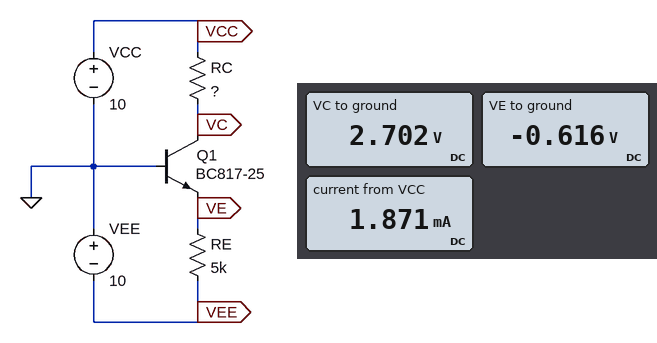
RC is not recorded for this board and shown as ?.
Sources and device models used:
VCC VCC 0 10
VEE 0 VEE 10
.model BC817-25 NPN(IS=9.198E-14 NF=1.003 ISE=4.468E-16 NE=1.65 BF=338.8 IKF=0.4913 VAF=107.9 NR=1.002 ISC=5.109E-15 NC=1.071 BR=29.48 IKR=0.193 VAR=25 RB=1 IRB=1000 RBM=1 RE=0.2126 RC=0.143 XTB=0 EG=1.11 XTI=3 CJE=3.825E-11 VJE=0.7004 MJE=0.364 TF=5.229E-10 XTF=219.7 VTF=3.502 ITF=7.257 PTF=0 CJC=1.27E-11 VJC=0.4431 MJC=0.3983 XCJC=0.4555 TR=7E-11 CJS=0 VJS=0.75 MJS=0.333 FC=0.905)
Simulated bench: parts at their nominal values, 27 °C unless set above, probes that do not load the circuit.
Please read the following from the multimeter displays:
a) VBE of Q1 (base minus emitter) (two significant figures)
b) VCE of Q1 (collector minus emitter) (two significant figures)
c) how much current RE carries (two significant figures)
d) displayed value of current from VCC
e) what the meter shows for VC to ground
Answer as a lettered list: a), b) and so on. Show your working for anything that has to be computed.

a) 0 V - (-616 mV) = 620 mV
b) 2.702 V - (-616 mV) = 3.3 V
c) (-616 mV - (-10 V)) / 5 kΩ = 1.9 mA
d) 1.871 mA
e) 2.702 V
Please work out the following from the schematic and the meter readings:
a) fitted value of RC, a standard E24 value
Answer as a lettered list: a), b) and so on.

a) 3.9 kΩ
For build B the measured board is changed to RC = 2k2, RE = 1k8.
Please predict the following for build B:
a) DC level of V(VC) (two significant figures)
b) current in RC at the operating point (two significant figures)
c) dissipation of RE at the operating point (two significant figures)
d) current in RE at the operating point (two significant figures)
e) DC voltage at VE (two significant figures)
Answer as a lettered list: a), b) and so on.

a) -650 mV
b) 4.8 mA
c) 48 mW
d) 5.2 mA
e) -670 mV
